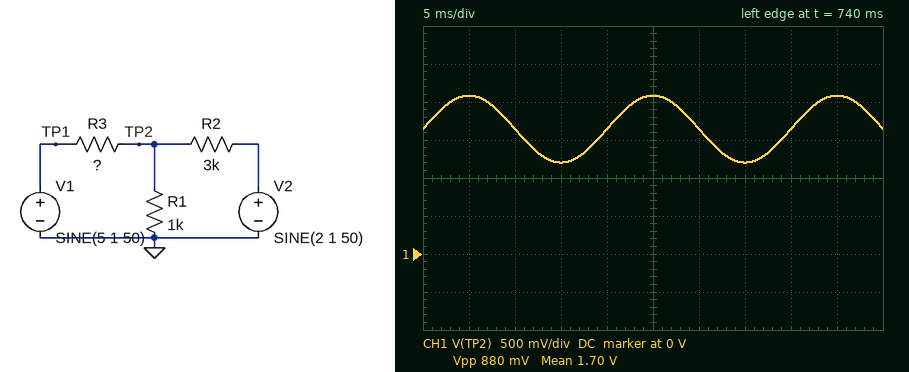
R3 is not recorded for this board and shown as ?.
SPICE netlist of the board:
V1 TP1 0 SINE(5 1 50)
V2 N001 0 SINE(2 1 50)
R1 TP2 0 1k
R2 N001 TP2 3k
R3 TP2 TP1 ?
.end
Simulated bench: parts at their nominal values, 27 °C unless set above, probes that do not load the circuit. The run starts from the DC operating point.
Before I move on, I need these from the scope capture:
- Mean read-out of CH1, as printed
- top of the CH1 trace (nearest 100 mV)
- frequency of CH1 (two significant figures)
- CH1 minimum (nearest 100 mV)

1.70 V
2.1 V
50 Hz
1.2 V
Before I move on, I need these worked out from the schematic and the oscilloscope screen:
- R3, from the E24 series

2.2 kΩ
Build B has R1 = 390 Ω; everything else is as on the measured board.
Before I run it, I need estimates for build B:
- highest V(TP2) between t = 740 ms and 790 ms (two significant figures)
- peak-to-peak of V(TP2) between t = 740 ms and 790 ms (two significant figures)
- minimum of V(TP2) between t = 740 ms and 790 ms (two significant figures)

1.1 V
470 mV
640 mV
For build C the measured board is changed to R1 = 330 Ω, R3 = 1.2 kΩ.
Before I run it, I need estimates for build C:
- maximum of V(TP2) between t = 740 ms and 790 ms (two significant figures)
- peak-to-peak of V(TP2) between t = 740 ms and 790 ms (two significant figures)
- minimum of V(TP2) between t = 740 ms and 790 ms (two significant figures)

1.4 V
560 mV
870 mV
